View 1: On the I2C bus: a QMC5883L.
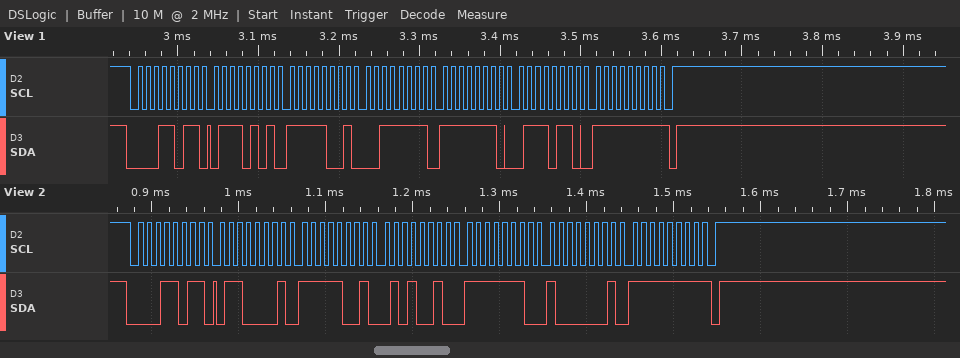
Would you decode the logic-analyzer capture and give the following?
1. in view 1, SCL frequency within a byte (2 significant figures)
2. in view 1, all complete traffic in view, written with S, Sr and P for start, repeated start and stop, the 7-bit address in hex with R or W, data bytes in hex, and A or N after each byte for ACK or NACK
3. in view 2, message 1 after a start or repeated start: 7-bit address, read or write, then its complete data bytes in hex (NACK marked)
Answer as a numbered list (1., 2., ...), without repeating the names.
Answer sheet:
1. 100 kHz
2. S 0DR A 75 A F9 A 3F A FE A 76 A FF N P
3. 0x0D read: 61 F9 52 FE 81 FF NACK
